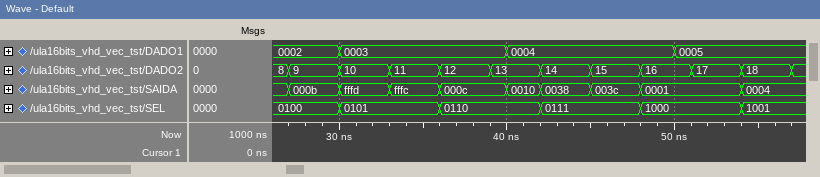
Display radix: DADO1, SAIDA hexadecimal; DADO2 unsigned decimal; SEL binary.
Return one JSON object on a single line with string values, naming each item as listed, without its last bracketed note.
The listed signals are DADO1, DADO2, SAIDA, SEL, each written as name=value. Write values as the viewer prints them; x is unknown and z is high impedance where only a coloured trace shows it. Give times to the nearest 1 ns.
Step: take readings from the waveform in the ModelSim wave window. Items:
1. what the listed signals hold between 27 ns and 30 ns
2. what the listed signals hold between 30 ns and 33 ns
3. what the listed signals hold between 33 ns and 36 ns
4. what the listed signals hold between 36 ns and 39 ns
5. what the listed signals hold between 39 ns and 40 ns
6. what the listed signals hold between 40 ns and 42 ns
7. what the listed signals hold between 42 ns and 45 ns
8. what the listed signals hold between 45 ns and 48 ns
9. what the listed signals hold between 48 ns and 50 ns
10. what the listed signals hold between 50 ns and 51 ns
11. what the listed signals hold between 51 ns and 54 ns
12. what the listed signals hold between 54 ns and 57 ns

{"what the listed signals hold between 27 ns and 30 ns": "DADO1=0002, DADO2=9, SAIDA=000b, SEL=0100", "what the listed signals hold between 30 ns and 33 ns": "DADO1=0003, DADO2=10, SAIDA=fffd, SEL=0101", "what the listed signals hold between 33 ns and 36 ns": "DADO1=0003, DADO2=11, SAIDA=fffc, SEL=0101", "what the listed signals hold between 36 ns and 39 ns": "DADO1=0003, DADO2=12, SAIDA=000c, SEL=0110", "what the listed signals hold between 39 ns and 40 ns": "DADO1=0003, DADO2=13, SAIDA=000c, SEL=0110", "what the listed signals hold between 40 ns and 42 ns": "DADO1=0004, DADO2=13, SAIDA=0010, SEL=0110", "what the listed signals hold between 42 ns and 45 ns": "DADO1=0004, DADO2=14, SAIDA=0038, SEL=0111", "what the listed signals hold between 45 ns and 48 ns": "DADO1=0004, DADO2=15, SAIDA=003c, SEL=0111", "what the listed signals hold between 48 ns and 50 ns": "DADO1=0004, DADO2=16, SAIDA=0001, SEL=1000", "what the listed signals hold between 50 ns and 51 ns": "DADO1=0005, DADO2=16, SAIDA=0001, SEL=1000", "what the listed signals hold between 51 ns and 54 ns": "DADO1=0005, DADO2=17, SAIDA=0001, SEL=1000", "what the listed signals hold between 54 ns and 57 ns": "DADO1=0005, DADO2=18, SAIDA=0004, SEL=1001"}
